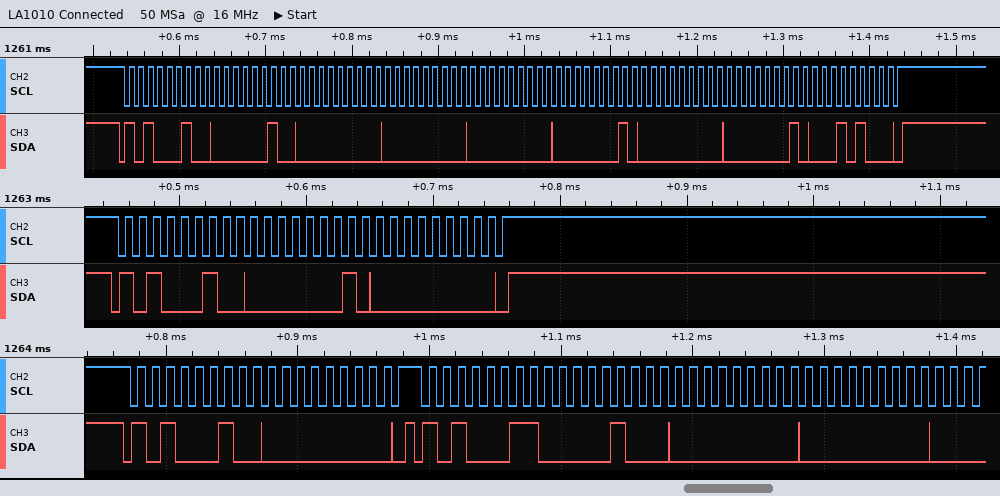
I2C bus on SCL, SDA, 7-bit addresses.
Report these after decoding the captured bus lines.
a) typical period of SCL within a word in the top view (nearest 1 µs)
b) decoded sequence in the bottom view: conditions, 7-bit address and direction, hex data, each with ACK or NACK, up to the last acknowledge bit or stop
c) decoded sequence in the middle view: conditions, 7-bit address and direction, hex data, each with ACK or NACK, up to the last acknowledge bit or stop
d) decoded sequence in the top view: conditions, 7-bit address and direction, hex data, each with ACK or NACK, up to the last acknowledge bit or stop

11 µs
start, address 51 write ACK, 00 ACK, stop, start, address 51 read ACK, 08 ACK, 00 ACK, 00 ACK
start, address 51 write ACK, 01 ACK, 00 ACK, stop
start, address 51 write ACK, 02 ACK, 00 ACK, 00 ACK, 00 ACK, 01 ACK, 00 ACK, 01 ACK, 14 ACK, stop
